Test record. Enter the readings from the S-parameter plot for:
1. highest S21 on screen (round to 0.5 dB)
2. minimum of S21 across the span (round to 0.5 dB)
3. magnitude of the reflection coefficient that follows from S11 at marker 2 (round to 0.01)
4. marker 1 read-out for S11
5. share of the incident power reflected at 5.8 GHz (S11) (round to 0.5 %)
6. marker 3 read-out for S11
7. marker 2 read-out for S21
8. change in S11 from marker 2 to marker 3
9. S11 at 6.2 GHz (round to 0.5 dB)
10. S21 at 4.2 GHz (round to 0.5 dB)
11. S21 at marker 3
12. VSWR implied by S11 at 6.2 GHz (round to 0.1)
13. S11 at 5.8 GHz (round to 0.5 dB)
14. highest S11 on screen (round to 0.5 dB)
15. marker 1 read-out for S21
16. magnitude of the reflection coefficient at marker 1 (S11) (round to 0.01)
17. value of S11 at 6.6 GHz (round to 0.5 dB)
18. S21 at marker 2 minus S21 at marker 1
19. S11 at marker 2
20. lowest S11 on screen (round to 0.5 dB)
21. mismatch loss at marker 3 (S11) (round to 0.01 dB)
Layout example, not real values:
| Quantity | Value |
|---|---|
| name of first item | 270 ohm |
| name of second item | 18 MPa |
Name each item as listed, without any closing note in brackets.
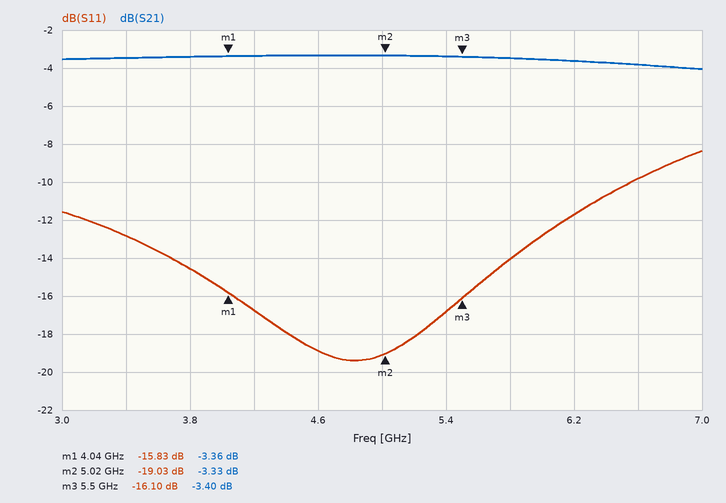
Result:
| Quantity | Value |
|---|---|
| highest S21 on screen | -3.5 dB |
| minimum of S21 across the span | -4.0 dB |
| magnitude of the reflection coefficient that follows from S11 at marker 2 | 0.11 |
| marker 1 read-out for S11 | -15.83 dB |
| share of the incident power reflected at 5.8 GHz (S11) | 4.0 % |
| marker 3 read-out for S11 | -16.10 dB |
| marker 2 read-out for S21 | -3.33 dB |
| change in S11 from marker 2 to marker 3 | 2.93 dB |
| S11 at 6.2 GHz | -11.5 dB |
| S21 at 4.2 GHz | -3.5 dB |
| S21 at marker 3 | -3.40 dB |
| VSWR implied by S11 at 6.2 GHz | 1.7 |
| S11 at 5.8 GHz | -14.0 dB |
| highest S11 on screen | -8.5 dB |
| marker 1 read-out for S21 | -3.36 dB |
| magnitude of the reflection coefficient at marker 1 (S11) | 0.16 |
| value of S11 at 6.6 GHz | -10.0 dB |
| S21 at marker 2 minus S21 at marker 1 | 0.03 dB |
| S11 at marker 2 | -19.03 dB |
| lowest S11 on screen | -19.5 dB |
| mismatch loss at marker 3 (S11) | 0.11 dB |
